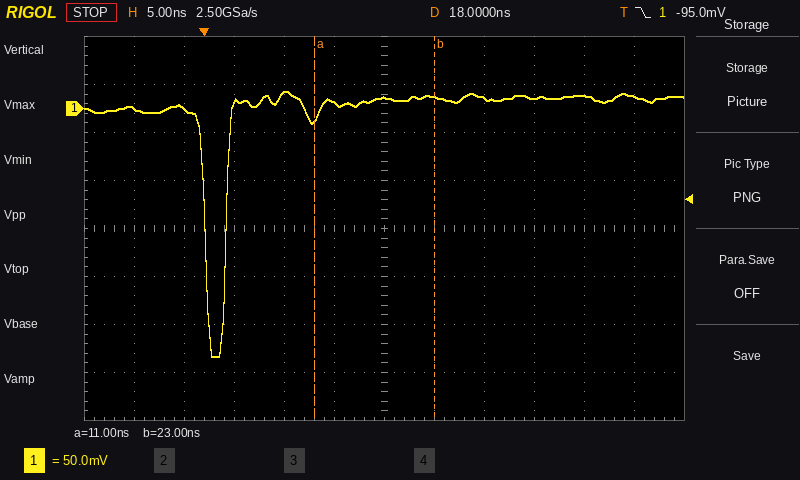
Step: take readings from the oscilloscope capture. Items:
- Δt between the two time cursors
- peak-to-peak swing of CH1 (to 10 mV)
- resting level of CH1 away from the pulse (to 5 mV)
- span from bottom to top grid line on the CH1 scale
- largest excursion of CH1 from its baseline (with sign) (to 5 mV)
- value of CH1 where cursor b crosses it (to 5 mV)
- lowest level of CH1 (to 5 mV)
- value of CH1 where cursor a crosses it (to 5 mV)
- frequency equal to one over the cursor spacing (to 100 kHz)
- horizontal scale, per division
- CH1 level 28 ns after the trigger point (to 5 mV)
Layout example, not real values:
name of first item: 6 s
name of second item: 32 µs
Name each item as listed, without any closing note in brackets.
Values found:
Δt between the two time cursors: 12.0 ns
peak-to-peak swing of CH1: 280 mV
resting level of CH1 away from the pulse: 10 mV
span from bottom to top grid line on the CH1 scale: 400 mV
largest excursion of CH1 from its baseline (with sign): -270 mV
value of CH1 where cursor b crosses it: 10 mV
lowest level of CH1: -260 mV
value of CH1 where cursor a crosses it: -10 mV
frequency equal to one over the cursor spacing: 83.3 MHz
horizontal scale, per division: 5 ns
CH1 level 28 ns after the trigger point: 10 mV
